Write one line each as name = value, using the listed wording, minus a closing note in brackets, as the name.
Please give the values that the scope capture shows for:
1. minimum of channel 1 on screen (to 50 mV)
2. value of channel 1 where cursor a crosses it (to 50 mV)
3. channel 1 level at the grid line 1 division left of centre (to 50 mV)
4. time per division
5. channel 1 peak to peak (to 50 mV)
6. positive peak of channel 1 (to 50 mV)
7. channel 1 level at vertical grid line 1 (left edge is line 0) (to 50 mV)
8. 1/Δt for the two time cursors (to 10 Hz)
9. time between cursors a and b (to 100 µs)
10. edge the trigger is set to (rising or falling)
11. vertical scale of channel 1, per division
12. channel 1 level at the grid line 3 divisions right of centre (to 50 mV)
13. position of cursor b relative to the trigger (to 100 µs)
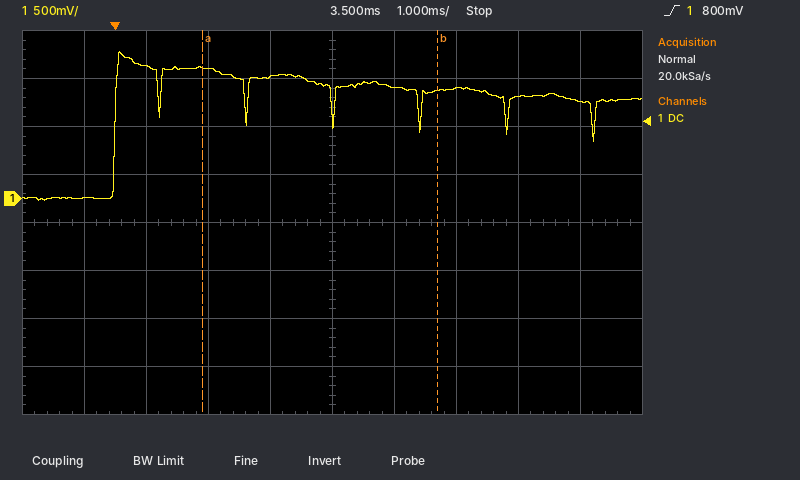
minimum of channel 1 on screen = 0 mV
value of channel 1 where cursor a crosses it = 1.35 V
channel 1 level at the grid line 1 division left of centre = 1.25 V
time per division = 1 ms
channel 1 peak to peak = 1.55 V
positive peak of channel 1 = 1.55 V
channel 1 level at vertical grid line 1 (left edge is line 0) = 0 mV
1/Δt for the two time cursors = 260 Hz
time between cursors a and b = 3.8 ms
edge the trigger is set to = rising
vertical scale of channel 1, per division = 500 mV
channel 1 level at the grid line 3 divisions right of centre = 1.05 V
position of cursor b relative to the trigger = +5.2 ms
